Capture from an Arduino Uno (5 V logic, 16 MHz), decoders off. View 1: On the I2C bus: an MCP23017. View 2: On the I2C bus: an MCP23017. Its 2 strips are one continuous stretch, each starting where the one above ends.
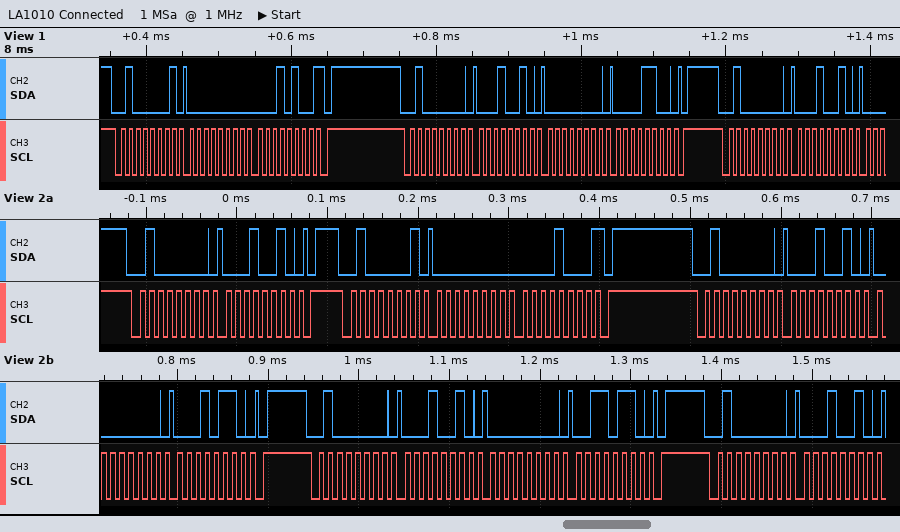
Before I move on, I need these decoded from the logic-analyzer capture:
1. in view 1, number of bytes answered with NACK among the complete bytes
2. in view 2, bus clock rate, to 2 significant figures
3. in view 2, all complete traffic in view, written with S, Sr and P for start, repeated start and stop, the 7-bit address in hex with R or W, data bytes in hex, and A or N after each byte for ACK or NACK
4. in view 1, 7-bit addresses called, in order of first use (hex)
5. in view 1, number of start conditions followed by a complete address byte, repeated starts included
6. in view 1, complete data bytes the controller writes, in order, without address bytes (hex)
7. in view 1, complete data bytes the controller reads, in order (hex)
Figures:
1
100 kHz
S 20W A 12 A P S 20R A 00 A 08 N P S 20W A 12 A 00 A 16 A P S 20W A 12 A 00 A 36 A P S 20W A 12 A
0x20
3
12 00 0C 12
00 14
